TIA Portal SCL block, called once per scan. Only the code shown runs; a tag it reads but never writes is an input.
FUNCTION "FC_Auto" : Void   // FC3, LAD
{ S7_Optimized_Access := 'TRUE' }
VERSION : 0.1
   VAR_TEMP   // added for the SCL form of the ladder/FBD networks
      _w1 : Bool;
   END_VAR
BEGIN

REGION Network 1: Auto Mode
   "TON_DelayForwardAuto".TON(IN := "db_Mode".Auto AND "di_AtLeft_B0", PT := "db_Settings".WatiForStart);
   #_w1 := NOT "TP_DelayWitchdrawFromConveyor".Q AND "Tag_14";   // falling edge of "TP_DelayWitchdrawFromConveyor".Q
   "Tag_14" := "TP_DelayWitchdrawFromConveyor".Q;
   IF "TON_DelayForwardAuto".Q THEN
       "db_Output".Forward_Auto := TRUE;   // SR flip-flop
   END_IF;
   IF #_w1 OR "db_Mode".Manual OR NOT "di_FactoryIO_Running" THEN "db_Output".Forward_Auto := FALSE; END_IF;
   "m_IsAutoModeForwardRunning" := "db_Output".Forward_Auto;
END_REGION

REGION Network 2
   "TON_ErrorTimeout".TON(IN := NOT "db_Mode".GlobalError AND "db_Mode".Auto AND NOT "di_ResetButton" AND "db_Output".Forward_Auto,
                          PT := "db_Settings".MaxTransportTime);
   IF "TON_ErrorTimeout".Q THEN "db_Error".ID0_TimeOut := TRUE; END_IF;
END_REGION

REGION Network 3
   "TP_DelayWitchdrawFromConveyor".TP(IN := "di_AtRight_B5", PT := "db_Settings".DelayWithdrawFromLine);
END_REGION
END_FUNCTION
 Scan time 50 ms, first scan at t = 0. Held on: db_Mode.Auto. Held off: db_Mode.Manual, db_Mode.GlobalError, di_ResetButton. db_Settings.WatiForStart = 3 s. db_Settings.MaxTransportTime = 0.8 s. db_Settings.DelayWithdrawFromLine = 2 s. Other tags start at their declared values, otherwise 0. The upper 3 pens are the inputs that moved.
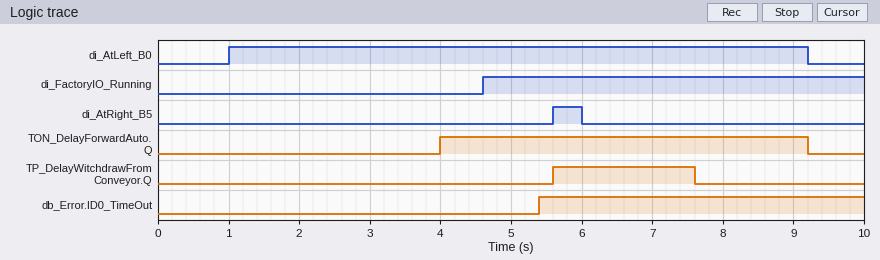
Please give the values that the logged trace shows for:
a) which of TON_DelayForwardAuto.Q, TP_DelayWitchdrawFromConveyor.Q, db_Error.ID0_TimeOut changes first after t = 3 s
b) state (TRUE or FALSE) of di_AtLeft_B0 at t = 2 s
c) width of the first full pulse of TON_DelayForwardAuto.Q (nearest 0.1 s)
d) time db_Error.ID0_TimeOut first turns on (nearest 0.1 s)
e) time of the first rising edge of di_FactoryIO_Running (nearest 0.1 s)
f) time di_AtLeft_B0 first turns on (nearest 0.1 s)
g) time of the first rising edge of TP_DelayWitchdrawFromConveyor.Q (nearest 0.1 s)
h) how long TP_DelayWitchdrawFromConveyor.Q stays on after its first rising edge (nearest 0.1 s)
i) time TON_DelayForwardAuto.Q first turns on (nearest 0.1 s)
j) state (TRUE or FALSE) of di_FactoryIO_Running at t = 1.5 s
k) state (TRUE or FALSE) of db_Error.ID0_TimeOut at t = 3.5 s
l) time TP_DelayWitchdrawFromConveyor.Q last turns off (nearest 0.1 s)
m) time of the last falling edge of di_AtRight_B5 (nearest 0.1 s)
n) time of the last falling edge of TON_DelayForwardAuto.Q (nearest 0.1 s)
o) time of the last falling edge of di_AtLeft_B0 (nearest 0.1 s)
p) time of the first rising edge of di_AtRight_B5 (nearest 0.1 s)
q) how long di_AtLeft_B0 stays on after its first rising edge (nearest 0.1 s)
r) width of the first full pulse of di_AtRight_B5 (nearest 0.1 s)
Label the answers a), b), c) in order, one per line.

a) TON_DelayForwardAuto.Q
b) TRUE
c) 5.2 s
d) 5.4 s
e) 4.6 s
f) 1.0 s
g) 5.6 s
h) 2.0 s
i) 4.0 s
j) FALSE
k) FALSE
l) 7.6 s
m) 6.0 s
n) 9.2 s
o) 9.2 s
p) 5.6 s
q) 8.2 s
r) 0.4 s
